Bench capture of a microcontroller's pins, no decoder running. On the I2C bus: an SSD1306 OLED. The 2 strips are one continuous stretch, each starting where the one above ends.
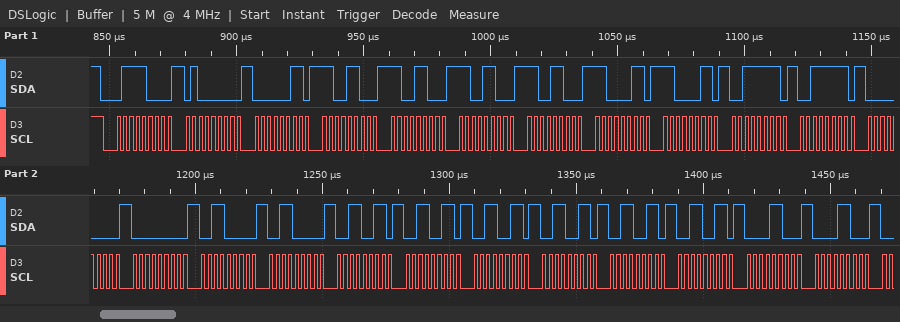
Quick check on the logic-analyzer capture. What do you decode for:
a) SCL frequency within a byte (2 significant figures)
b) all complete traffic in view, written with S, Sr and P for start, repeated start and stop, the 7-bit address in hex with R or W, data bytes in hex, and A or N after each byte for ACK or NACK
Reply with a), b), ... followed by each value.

a) 400 kHz
b) S 3CW A 40 A 03 A CC A CC A CC A CC A C3 A C3 A 3F A 3F A 00 A 00 A 30 A 30 A 33 A 33 A 33 A 33 A 33 A 33 A 0C A 0C A
